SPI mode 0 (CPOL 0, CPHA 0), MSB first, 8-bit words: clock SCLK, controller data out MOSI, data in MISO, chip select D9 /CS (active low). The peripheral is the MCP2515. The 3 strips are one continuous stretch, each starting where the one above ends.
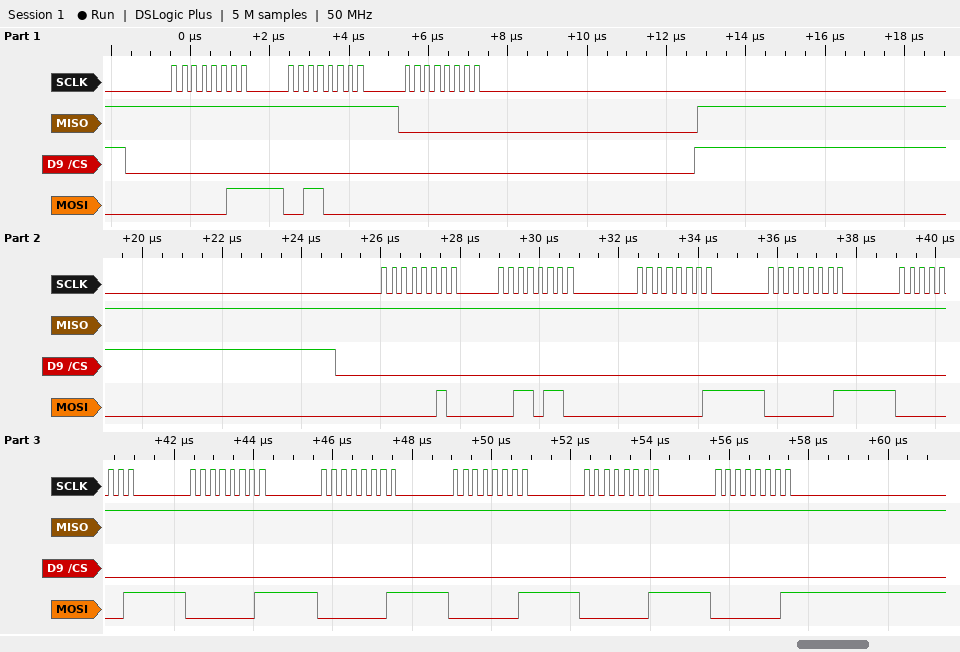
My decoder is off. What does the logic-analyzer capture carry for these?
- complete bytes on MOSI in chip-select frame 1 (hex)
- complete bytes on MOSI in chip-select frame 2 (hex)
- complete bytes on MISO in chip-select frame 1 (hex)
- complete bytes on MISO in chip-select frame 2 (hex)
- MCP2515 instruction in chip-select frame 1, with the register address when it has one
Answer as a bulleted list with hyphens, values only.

- 0x03 0x30 0x00
- 0x02 0x36 0x01 0x01 0x01 0x01 0x01 0x01 0x01 0x01
- 0xFF 0xFF 0x00
- 0xFF 0xFF 0xFF 0xFF 0xFF 0xFF 0xFF 0xFF 0xFF 0xFF
- READ 0x30
